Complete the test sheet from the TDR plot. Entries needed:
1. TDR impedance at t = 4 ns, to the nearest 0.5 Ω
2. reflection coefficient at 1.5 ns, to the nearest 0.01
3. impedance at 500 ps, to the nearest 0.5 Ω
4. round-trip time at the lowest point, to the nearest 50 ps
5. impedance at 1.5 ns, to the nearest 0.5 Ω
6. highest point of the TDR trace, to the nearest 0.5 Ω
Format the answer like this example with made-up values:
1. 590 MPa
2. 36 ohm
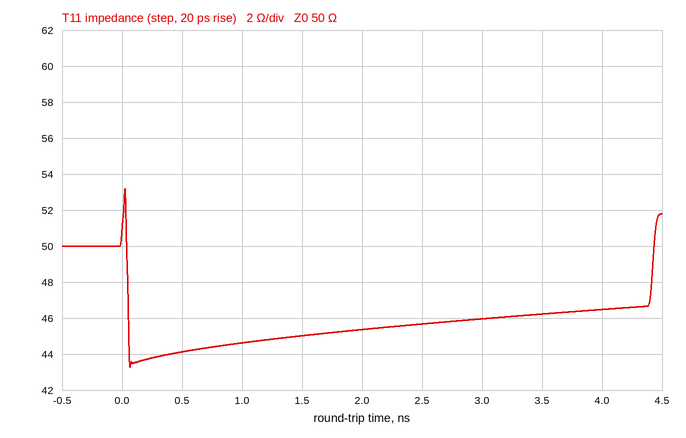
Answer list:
1. 46.5 Ω
2. -0.05
3. 44.0 Ω
4. 50 ps
5. 45.0 Ω
6. 53.0 Ω
